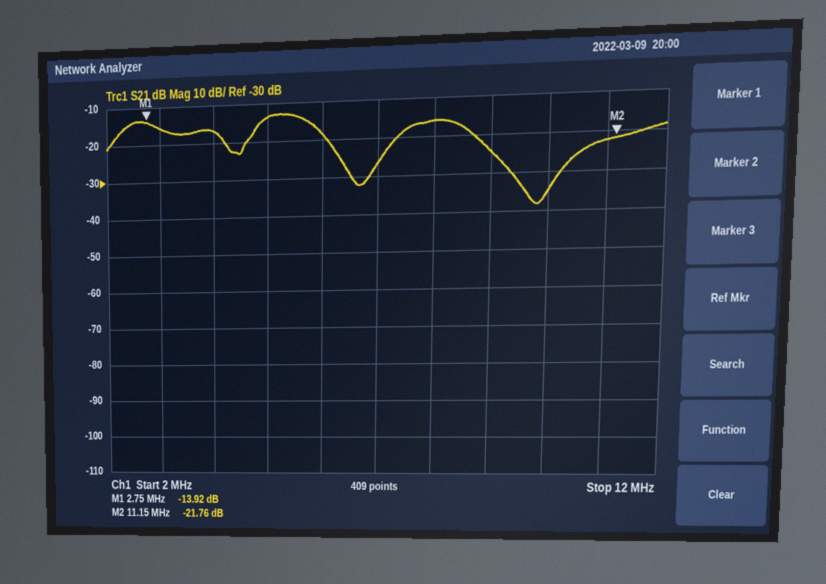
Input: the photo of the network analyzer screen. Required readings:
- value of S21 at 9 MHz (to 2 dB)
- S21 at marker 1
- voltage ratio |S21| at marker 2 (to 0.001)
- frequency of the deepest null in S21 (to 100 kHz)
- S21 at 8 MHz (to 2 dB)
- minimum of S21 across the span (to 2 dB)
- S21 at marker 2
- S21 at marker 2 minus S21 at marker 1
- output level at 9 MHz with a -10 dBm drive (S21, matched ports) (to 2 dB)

-24 dB
-13.92 dB
0.082
9.8 MHz
-16 dB
-38 dB
-21.76 dB
-7.84 dB
-34 dBm
